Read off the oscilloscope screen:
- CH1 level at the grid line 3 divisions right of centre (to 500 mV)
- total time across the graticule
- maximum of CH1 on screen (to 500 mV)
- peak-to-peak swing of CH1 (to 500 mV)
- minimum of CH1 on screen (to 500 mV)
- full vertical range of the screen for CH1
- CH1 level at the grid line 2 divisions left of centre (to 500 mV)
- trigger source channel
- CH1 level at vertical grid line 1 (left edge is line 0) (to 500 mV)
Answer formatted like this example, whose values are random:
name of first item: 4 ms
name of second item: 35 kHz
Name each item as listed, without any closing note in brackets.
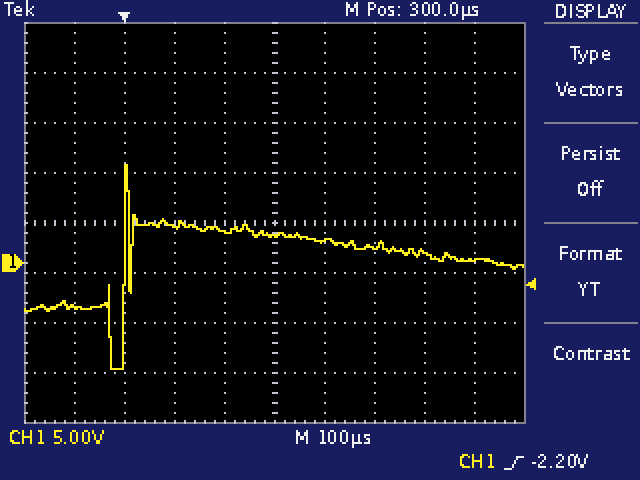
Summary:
CH1 level at the grid line 3 divisions right of centre: 1.0 V
total time across the graticule: 1 ms
maximum of CH1 on screen: 10.0 V
peak-to-peak swing of CH1: 20.5 V
minimum of CH1 on screen: -10.5 V
full vertical range of the screen for CH1: 40 V
CH1 level at the grid line 2 divisions left of centre: 3.5 V
trigger source channel: CH1
CH1 level at vertical grid line 1 (left edge is line 0): -4.5 V
